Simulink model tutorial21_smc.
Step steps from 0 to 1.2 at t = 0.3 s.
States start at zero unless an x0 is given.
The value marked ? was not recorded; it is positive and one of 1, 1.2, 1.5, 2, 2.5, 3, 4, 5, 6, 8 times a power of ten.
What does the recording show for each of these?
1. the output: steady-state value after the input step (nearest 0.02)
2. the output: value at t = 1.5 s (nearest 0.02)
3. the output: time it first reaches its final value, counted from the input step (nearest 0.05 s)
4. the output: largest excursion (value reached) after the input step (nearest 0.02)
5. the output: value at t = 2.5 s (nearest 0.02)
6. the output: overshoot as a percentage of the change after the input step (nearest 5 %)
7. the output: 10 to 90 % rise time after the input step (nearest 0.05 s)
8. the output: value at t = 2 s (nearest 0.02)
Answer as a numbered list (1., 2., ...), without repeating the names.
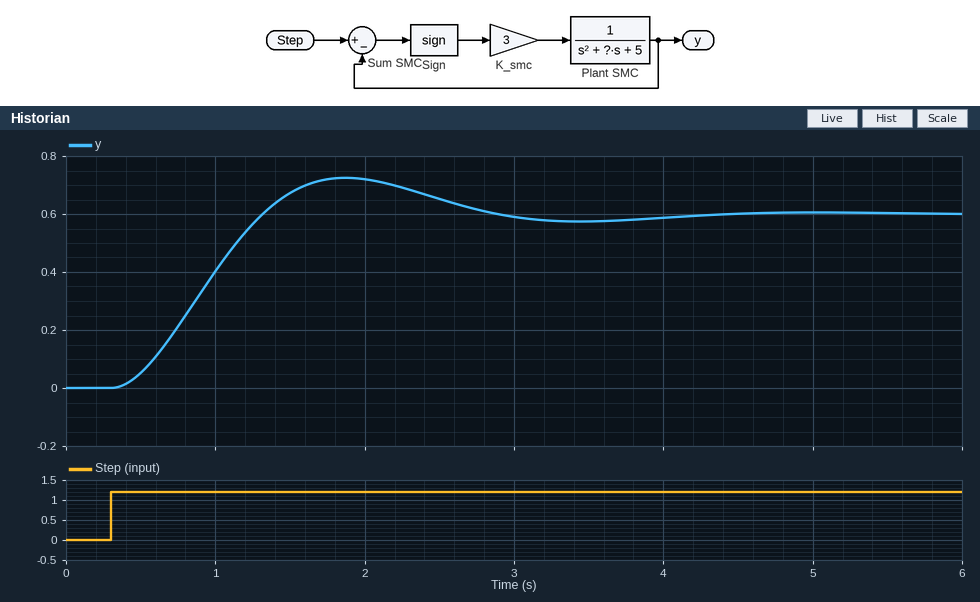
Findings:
1. 0.60
2. 0.68
3. 1.00 s
4. 0.72
5. 0.66
6. 20 %
7. 0.70 s
8. 0.72
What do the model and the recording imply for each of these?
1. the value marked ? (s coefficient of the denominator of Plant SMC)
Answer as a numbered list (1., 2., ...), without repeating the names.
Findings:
1. 2
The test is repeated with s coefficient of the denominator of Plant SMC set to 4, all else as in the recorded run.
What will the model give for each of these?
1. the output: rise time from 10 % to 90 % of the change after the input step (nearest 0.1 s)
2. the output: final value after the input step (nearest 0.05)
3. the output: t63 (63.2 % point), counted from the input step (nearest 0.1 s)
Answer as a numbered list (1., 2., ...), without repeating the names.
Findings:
1. 1.3 s
2. 0.60
3. 0.9 s
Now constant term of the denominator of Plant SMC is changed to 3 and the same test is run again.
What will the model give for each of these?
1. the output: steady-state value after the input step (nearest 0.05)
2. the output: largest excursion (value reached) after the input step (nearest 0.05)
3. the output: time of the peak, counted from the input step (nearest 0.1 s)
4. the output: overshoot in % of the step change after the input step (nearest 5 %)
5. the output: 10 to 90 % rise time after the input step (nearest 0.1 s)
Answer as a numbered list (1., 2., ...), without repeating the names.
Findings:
1. 1.00
2. 1.10
3. 2.2 s
4. 10 %
5. 1.0 s
